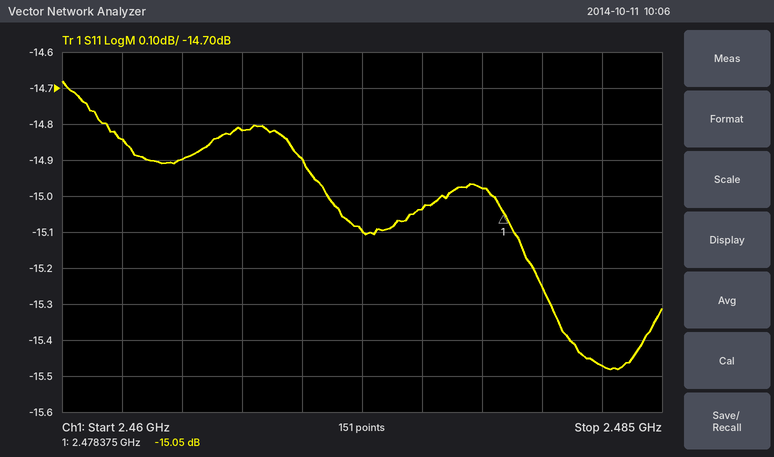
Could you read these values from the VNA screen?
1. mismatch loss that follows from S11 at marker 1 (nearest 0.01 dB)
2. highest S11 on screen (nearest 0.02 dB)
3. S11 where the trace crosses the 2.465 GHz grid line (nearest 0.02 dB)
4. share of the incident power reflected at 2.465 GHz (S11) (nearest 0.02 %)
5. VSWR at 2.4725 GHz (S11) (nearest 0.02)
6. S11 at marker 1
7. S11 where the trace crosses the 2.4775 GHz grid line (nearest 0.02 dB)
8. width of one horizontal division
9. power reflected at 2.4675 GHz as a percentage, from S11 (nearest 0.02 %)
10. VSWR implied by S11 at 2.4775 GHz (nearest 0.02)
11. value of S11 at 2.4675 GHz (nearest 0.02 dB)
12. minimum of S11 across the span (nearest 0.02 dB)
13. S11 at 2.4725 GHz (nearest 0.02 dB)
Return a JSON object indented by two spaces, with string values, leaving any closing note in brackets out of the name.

{
  "mismatch loss that follows from S11 at marker 1": "0.14 dB",
  "highest S11 on screen": "-14.68 dB",
  "S11 where the trace crosses the 2.465 GHz grid line": "-14.90 dB",
  "share of the incident power reflected at 2.465 GHz (S11)": "3.24 %",
  "VSWR at 2.4725 GHz (S11)": "1.42",
  "S11 at marker 1": "-15.05 dB",
  "S11 where the trace crosses the 2.4775 GHz grid line": "-14.98 dB",
  "width of one horizontal division": "2.5 MHz",
  "power reflected at 2.4675 GHz as a percentage, from S11": "3.30 %",
  "VSWR implied by S11 at 2.4775 GHz": "1.44",
  "value of S11 at 2.4675 GHz": "-14.82 dB",
  "minimum of S11 across the span": "-15.48 dB",
  "S11 at 2.4725 GHz": "-15.10 dB"
}
